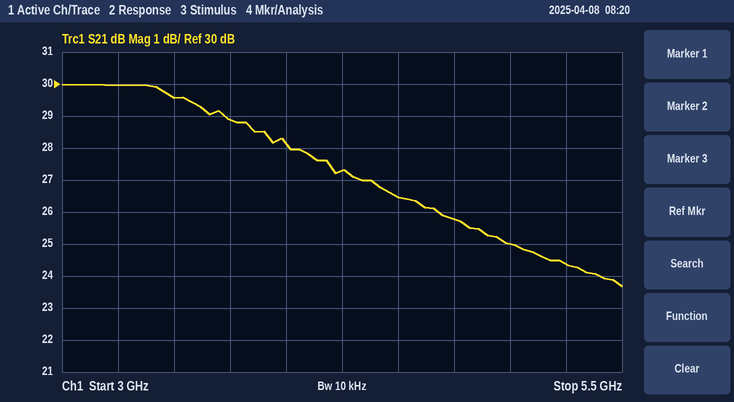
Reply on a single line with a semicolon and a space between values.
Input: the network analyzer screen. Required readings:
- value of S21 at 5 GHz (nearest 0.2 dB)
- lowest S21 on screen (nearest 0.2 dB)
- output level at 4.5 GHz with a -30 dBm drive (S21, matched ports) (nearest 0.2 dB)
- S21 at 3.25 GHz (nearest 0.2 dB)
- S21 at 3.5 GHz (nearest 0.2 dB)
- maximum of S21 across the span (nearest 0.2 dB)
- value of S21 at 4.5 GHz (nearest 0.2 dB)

25.0 dB; 23.6 dB; -3.6 dBm; 30.0 dB; 29.6 dB; 30.0 dB; 26.4 dB
